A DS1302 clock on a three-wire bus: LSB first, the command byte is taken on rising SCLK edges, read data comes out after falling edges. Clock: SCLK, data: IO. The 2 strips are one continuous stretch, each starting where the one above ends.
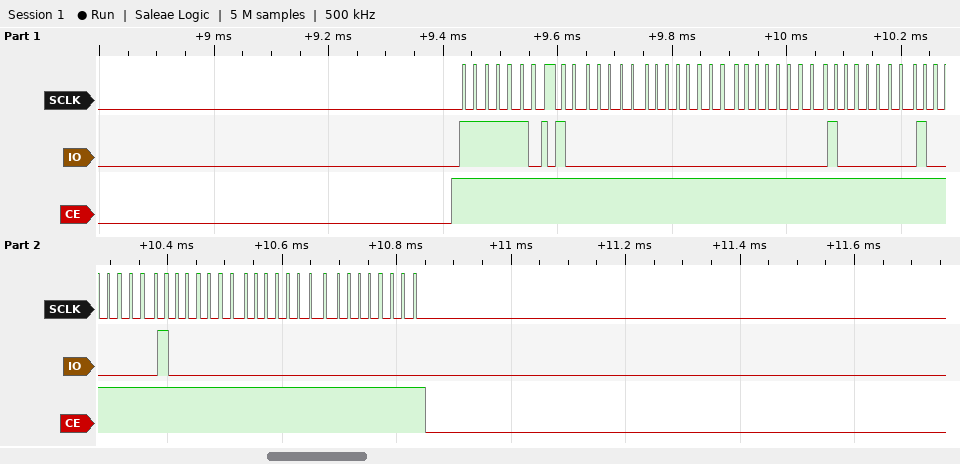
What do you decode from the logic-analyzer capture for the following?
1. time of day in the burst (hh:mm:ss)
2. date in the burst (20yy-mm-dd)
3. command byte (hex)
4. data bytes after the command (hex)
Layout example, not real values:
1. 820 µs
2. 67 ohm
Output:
1. 00:00:01
2. 2000-01-01
3. 0xBF
4. 01 00 00 01 01 01 00 00
